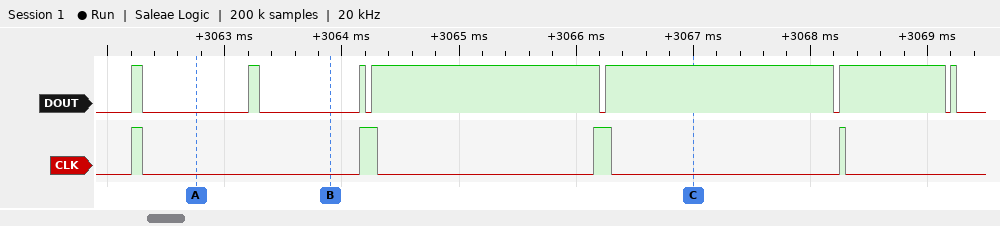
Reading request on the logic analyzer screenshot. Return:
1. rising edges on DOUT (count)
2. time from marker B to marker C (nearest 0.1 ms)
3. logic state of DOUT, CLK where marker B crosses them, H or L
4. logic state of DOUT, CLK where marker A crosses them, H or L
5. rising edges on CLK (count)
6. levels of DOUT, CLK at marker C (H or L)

7
3.1 ms
DOUT=L, CLK=L
DOUT=L, CLK=L
4
DOUT=H, CLK=L
